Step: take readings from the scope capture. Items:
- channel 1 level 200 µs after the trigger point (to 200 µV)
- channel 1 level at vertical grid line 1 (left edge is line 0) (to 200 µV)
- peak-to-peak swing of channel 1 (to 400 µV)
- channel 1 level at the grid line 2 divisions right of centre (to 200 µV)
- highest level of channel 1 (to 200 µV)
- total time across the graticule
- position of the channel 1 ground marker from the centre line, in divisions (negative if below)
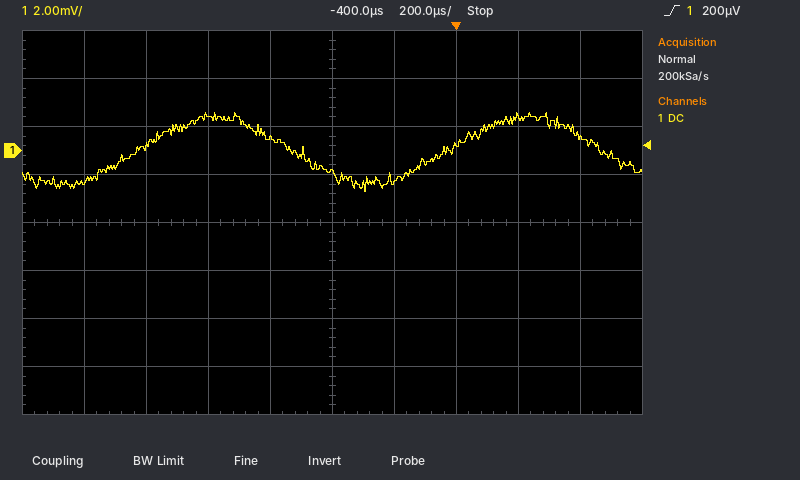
1.4 mV
-1.2 mV
3.2 mV
200 µV
1.6 mV
2 ms
+1.5 div
